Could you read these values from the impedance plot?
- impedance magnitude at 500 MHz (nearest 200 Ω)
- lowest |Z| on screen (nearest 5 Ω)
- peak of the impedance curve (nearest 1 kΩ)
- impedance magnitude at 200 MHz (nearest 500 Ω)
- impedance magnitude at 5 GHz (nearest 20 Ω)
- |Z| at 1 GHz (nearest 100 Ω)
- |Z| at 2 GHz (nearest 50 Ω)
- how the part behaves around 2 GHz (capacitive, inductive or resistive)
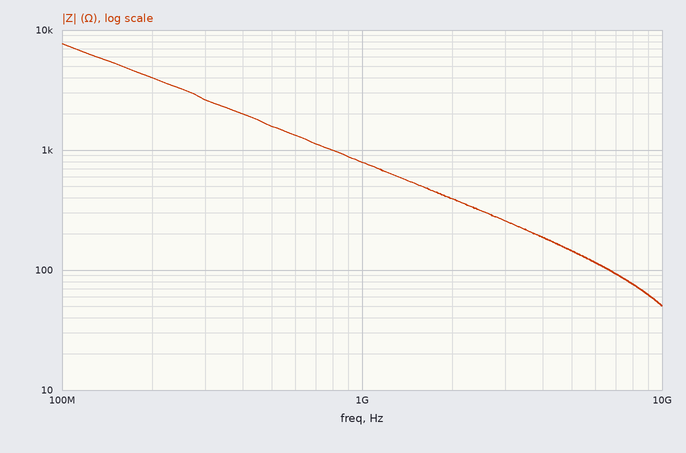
1.6 kΩ
50 Ω
8 kΩ
4.0 kΩ
140 Ω
800 Ω
400 Ω
capacitive
